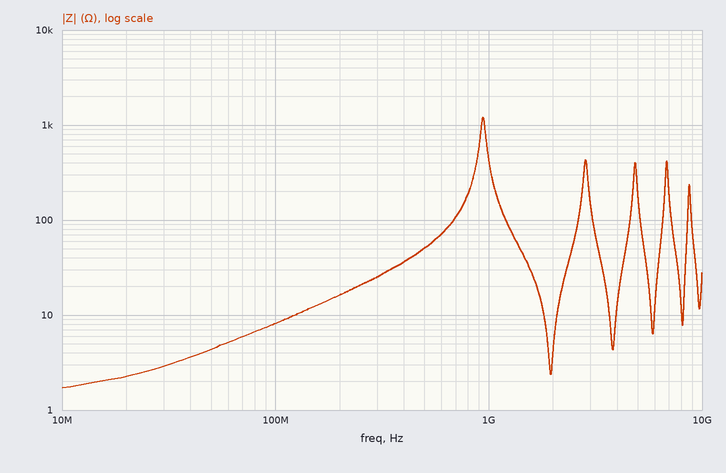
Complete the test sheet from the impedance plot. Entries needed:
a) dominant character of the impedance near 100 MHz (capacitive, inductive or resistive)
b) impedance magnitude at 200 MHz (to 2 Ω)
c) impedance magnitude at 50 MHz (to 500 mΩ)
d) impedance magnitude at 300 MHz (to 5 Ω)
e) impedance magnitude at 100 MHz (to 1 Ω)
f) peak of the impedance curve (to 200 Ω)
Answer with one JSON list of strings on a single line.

["inductive", "16 Ω", "4.5 Ω", "25 Ω", "8 Ω", "1.2 kΩ"]
